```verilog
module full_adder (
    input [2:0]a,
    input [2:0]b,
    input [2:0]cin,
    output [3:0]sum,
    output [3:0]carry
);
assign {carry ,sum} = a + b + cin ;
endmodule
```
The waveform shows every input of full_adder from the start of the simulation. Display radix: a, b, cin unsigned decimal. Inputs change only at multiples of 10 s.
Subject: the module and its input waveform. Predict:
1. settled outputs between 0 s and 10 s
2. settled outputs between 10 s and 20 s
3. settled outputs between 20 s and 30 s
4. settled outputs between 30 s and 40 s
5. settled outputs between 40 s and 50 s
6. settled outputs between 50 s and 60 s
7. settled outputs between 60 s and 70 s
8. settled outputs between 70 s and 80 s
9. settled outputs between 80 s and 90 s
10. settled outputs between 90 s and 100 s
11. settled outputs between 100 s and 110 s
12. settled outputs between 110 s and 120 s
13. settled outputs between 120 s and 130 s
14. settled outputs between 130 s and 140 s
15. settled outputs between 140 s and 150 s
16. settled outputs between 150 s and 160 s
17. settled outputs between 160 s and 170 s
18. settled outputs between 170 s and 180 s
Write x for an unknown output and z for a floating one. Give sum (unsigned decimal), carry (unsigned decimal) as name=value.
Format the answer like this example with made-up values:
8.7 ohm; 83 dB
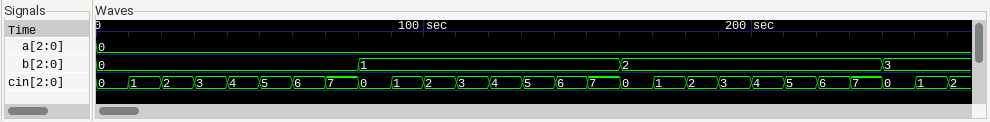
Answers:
sum=0, carry=0; sum=1, carry=0; sum=2, carry=0; sum=3, carry=0; sum=4, carry=0; sum=5, carry=0; sum=6, carry=0; sum=7, carry=0; sum=1, carry=0; sum=2, carry=0; sum=3, carry=0; sum=4, carry=0; sum=5, carry=0; sum=6, carry=0; sum=7, carry=0; sum=8, carry=0; sum=2, carry=0; sum=3, carry=0
